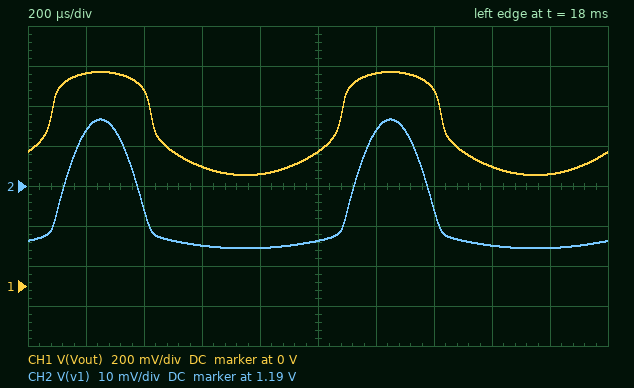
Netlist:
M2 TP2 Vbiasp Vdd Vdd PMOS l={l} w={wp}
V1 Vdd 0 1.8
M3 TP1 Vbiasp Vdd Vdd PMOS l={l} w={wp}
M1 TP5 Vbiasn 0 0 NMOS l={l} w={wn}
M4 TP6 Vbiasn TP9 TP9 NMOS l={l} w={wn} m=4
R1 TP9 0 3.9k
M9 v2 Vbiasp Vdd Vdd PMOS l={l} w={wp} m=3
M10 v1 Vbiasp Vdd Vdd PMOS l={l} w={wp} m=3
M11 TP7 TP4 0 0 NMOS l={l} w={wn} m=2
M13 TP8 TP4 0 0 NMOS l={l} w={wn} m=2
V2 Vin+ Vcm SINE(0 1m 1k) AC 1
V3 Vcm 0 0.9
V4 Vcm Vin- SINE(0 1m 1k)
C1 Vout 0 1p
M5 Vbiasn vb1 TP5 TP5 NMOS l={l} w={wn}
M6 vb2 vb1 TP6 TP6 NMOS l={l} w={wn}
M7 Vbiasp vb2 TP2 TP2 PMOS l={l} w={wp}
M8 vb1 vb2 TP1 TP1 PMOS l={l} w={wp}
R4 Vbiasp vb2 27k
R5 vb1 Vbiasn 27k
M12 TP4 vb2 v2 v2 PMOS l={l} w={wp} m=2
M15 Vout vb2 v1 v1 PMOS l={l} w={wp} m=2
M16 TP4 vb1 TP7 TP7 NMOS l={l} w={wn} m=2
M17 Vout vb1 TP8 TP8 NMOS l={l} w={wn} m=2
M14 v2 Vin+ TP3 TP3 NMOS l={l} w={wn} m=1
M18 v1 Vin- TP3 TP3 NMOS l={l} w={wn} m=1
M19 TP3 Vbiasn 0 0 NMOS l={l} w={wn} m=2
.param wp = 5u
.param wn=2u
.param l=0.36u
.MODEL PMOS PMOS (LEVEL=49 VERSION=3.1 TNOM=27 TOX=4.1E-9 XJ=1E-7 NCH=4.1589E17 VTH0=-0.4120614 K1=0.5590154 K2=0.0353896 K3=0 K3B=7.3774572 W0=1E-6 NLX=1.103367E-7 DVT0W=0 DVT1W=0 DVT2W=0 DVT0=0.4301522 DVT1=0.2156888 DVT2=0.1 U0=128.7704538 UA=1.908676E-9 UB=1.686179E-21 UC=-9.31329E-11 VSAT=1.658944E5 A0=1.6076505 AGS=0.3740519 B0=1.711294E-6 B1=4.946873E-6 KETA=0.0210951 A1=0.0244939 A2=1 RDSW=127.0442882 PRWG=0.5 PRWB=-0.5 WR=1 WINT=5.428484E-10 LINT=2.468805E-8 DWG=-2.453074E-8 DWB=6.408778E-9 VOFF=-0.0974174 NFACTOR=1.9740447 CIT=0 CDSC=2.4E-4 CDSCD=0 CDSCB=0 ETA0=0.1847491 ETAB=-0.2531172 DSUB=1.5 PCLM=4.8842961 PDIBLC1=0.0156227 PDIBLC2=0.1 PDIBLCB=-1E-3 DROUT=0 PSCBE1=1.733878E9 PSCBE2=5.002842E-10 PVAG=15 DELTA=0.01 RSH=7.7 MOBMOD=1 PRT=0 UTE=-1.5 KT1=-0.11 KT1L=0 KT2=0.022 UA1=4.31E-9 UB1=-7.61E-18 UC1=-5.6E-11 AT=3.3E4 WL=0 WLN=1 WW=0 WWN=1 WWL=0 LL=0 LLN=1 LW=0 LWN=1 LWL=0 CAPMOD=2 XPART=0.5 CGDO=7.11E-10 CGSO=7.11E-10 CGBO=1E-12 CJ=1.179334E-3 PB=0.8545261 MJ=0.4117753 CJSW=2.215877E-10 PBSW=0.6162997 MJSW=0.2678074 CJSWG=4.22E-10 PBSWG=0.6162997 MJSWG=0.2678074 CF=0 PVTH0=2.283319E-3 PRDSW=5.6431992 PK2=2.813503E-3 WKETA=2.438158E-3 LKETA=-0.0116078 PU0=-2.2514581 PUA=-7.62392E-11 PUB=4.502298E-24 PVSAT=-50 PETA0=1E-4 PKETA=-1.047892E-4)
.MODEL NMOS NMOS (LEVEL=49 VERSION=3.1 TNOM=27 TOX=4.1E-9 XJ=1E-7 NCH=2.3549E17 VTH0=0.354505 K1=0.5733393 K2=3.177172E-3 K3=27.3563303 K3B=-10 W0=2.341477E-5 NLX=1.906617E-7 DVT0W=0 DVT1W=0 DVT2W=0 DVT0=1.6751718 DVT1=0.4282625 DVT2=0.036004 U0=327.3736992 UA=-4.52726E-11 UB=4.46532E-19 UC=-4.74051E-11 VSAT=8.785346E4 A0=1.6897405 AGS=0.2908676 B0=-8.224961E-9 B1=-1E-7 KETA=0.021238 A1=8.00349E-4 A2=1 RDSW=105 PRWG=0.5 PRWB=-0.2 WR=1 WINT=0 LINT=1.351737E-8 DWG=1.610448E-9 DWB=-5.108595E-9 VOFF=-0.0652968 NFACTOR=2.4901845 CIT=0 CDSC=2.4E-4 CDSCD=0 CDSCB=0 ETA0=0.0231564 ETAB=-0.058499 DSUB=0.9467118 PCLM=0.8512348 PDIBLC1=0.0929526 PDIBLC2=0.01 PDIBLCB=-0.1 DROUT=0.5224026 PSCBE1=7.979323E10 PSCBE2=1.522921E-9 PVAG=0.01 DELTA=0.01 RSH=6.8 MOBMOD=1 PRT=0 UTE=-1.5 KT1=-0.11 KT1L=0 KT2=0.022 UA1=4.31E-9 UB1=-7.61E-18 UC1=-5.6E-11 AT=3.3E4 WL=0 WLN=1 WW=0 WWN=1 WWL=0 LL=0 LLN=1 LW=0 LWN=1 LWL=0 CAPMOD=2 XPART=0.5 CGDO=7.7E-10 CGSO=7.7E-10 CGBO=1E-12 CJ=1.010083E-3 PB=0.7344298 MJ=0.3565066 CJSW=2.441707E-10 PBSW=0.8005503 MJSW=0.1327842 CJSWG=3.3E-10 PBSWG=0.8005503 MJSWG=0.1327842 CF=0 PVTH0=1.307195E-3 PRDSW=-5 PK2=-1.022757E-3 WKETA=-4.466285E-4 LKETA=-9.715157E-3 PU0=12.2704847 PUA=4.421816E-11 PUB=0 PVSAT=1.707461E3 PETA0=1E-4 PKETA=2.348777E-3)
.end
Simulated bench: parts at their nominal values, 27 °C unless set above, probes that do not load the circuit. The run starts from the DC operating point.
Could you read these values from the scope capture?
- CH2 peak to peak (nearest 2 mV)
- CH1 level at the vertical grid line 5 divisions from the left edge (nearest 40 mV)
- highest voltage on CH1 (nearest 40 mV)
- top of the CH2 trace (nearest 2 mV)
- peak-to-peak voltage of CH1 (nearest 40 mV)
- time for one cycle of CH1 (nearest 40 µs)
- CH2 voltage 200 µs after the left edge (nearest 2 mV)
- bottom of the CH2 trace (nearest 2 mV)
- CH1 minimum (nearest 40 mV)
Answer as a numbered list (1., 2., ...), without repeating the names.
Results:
1. 32 mV
2. 680 mV
3. 1.08 V
4. 1.206 V
5. 520 mV
6. 1.00 ms
7. 1.204 V
8. 1.174 V
9. 560 mV
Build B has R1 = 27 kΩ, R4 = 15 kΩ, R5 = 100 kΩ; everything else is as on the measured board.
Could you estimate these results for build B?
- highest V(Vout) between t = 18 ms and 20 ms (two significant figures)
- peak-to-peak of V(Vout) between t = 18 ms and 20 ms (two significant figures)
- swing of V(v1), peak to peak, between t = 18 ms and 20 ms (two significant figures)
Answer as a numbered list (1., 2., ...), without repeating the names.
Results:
1. 810 mV
2. 530 mV
3. 2.1 mV
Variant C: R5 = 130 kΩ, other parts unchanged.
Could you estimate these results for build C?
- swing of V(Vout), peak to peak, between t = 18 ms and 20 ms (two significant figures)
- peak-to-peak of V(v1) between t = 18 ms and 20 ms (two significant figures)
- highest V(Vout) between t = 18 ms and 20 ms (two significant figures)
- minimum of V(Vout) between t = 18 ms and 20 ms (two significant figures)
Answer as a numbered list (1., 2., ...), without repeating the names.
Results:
1. 130 mV
2. 1.9 mV
3. 700 mV
4. 570 mV
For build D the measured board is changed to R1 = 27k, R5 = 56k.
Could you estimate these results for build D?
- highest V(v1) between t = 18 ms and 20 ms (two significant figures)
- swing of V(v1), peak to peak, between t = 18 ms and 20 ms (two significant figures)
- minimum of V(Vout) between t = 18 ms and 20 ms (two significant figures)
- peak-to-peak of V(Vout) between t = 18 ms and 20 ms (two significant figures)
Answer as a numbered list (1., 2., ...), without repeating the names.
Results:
1. 1.7 V
2. 4.2 mV
3. 170 mV
4. 920 mV
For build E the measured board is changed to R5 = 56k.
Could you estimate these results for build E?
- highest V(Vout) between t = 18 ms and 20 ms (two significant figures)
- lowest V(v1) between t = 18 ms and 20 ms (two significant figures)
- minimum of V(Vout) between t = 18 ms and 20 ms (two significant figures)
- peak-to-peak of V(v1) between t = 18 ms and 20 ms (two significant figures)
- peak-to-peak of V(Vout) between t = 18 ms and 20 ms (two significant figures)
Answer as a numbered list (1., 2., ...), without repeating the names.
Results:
1. 750 mV
2. 1.3 V
3. 580 mV
4. 2.9 mV
5. 170 mV
